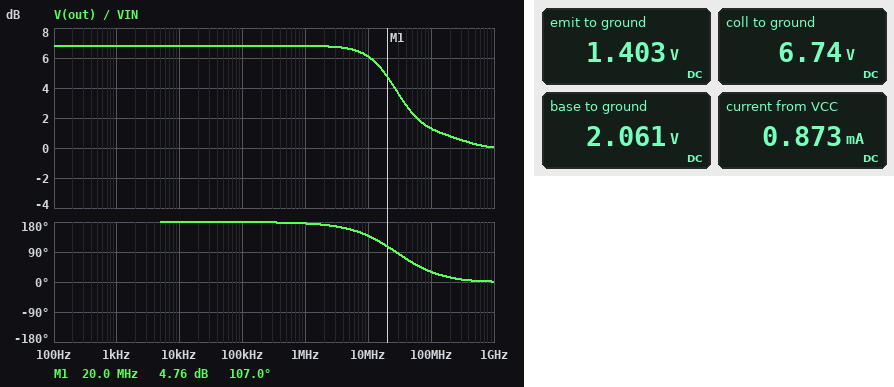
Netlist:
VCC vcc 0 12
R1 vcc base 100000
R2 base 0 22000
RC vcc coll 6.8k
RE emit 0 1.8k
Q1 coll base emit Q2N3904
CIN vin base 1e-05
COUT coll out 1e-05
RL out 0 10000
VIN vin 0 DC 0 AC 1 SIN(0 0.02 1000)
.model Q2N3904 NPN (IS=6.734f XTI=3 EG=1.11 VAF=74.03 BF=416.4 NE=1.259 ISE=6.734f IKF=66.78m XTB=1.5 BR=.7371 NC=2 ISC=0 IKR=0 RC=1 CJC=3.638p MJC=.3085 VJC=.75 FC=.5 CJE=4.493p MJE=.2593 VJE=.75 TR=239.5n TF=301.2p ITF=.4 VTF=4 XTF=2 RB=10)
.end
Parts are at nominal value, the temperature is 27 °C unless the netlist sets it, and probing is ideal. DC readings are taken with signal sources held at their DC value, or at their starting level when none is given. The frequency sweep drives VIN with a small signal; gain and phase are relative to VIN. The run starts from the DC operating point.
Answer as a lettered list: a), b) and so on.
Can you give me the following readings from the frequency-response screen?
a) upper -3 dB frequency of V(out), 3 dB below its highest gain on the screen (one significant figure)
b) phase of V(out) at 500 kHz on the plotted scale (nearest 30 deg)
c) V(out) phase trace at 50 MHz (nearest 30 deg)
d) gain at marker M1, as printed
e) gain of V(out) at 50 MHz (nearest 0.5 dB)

a) 30 MHz
b) 180 deg
c) 60 deg
d) 4.76 dB
e) 2.5 dB
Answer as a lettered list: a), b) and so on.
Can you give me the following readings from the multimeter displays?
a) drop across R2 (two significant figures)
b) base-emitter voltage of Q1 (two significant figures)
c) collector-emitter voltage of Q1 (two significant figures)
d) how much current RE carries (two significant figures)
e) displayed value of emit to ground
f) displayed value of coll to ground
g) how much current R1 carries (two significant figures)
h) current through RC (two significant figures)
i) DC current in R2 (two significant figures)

a) 2.1 V
b) 660 mV
c) 5.3 V
d) 780 µA
e) 1.403 V
f) 6.74 V
g) 99 µA
h) 770 µA
i) 94 µA
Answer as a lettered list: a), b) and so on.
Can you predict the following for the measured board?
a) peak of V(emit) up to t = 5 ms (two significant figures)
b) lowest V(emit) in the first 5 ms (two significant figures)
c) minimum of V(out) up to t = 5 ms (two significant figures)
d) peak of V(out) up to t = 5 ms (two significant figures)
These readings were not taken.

a) 1.4 V
b) 1.4 V
c) -44 mV
d) 44 mV
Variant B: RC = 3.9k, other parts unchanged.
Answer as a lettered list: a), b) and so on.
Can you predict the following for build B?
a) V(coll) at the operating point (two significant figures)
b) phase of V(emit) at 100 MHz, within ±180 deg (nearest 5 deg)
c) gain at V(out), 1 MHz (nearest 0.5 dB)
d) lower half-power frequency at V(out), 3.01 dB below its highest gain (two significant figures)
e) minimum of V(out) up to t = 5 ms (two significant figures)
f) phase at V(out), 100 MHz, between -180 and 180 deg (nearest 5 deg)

a) 9.0 V
b) 0 deg
c) 3.5 dB
d) 1.6 Hz
e) -30 mV
f) 40 deg
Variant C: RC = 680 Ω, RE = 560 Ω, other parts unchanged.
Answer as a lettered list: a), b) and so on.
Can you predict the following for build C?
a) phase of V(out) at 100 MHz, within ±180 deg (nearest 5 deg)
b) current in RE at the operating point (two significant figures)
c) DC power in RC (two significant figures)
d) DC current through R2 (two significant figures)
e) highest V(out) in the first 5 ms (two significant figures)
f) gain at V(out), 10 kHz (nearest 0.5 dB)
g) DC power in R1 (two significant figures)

a) 105 deg
b) 2.2 mA
c) 3.3 mW
d) 87 µA
e) 22 mV
f) 1.0 dB
g) 1.0 mW
